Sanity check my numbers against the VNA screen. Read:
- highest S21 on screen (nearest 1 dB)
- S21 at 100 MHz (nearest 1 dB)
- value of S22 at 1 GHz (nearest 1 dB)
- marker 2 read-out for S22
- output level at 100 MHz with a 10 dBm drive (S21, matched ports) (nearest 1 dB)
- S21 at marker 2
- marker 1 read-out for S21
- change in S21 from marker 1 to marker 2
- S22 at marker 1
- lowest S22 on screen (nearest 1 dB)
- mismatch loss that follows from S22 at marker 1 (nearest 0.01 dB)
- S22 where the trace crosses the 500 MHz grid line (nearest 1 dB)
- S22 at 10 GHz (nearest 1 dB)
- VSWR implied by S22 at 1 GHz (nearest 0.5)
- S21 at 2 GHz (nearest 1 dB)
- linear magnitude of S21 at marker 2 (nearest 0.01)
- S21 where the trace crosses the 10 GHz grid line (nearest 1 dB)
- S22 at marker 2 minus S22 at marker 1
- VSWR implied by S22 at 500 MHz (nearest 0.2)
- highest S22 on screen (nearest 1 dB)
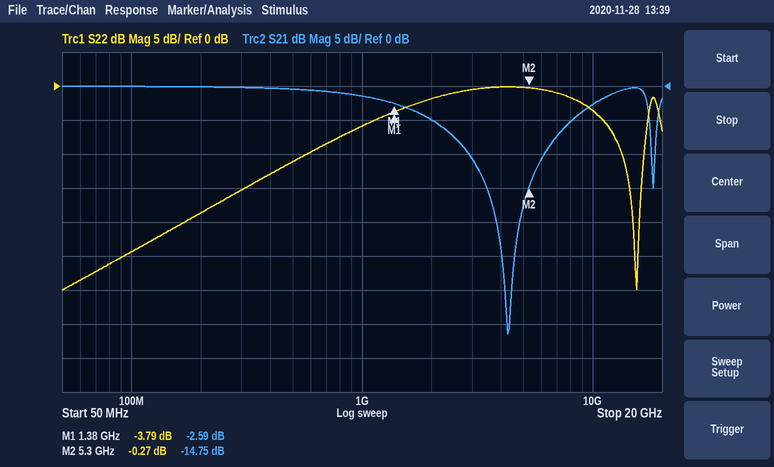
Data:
0 dB
0 dB
-6 dB
-0.27 dB
10 dBm
-14.75 dB
-2.59 dB
-12.16 dB
-3.79 dB
-30 dB
2.35 dB
-11 dB
-4 dB
3.0
-5 dB
0.18
-3 dB
3.52 dB
1.8
0 dB
